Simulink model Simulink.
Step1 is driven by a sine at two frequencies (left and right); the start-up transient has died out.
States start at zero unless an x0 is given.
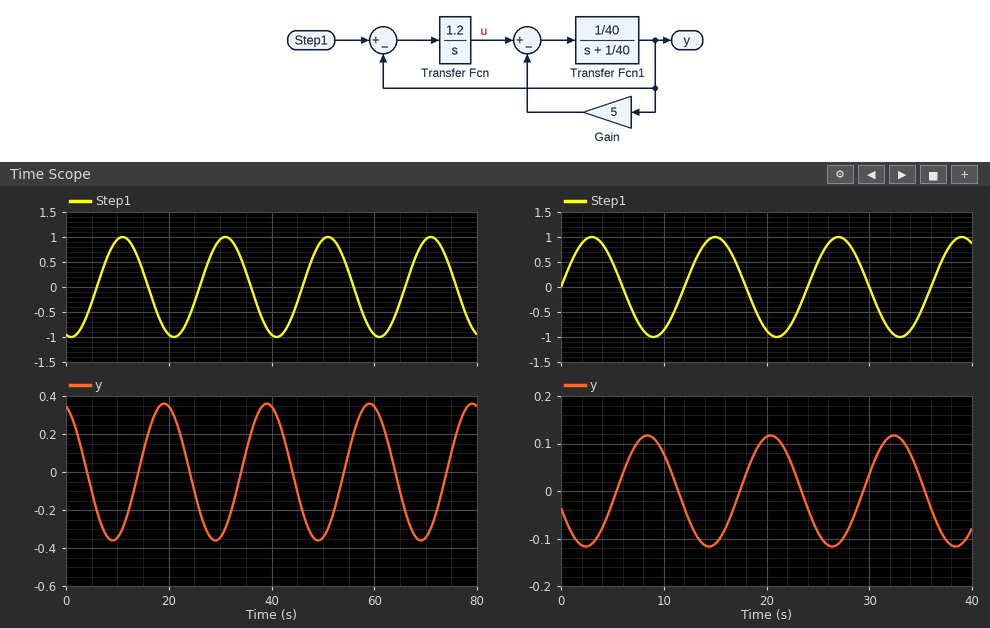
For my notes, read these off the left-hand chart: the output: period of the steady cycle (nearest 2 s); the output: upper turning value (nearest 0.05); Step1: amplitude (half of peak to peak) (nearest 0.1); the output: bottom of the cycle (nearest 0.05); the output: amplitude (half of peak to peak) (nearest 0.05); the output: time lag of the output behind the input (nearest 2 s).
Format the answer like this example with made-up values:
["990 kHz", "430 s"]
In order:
["20 s", "0.35", "1.0", "-0.35", "0.35", "8 s"]
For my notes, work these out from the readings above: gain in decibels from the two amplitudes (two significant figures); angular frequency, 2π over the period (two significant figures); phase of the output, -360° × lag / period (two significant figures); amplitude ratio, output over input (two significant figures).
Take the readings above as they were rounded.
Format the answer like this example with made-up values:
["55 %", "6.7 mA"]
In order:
["-9.1 dB", "0.31 rad/s", "-140°", "0.35"]
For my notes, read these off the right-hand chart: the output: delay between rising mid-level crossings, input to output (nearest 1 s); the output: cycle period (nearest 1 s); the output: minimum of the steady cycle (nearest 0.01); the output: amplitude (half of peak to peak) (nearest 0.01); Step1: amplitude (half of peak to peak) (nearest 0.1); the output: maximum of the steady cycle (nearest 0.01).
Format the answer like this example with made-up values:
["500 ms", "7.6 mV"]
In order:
["5 s", "12 s", "-0.12", "0.12", "1.0", "0.12"]
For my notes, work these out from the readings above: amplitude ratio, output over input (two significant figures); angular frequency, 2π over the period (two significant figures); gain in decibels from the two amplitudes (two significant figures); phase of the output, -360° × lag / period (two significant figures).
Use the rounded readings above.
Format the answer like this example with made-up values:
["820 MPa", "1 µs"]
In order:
["0.12", "0.52 rad/s", "-18 dB", "-150°"]
